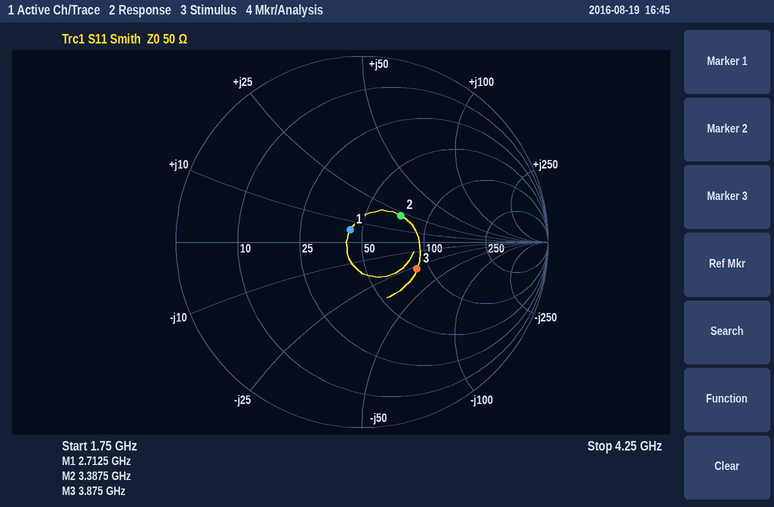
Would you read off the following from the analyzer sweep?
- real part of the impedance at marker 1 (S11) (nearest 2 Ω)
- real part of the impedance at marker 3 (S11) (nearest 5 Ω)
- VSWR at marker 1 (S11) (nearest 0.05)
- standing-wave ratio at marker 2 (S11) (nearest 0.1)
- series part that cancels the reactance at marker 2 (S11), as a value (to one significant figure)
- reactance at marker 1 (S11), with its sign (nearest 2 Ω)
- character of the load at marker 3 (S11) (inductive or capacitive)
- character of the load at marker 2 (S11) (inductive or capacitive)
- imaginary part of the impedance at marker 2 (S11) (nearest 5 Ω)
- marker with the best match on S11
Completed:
44 Ω
85 Ω
1.20
1.7
2 pF
+6 Ω
capacitive
inductive
+20 Ω
marker 1
